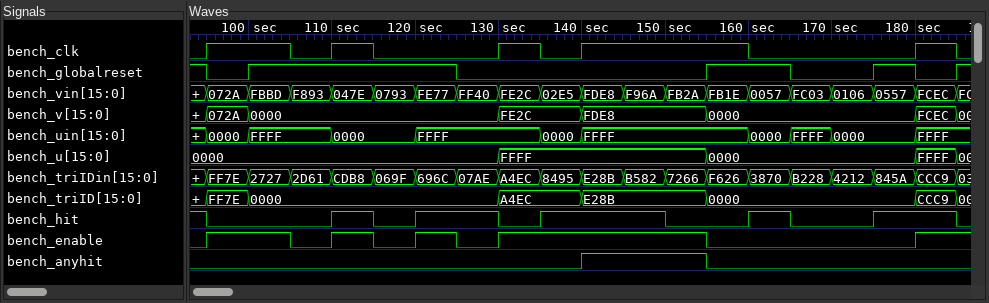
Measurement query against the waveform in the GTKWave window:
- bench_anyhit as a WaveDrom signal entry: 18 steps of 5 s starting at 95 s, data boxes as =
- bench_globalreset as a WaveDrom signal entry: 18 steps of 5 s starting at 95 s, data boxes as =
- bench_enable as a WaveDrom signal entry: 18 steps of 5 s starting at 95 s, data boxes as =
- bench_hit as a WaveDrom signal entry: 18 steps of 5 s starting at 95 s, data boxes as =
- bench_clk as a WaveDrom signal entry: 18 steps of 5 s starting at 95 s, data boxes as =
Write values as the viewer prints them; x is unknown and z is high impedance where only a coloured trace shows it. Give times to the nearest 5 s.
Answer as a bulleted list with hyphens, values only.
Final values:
- {name: 'bench_anyhit', wave: '0........1..0.....'}
- {name: 'bench_globalreset', wave: '01....0.....1.0.10'}
- {name: 'bench_enable', wave: '1.010101....0....1'}
- {name: 'bench_hit', wave: '0..101.01..0.10.1.'}
- {name: 'bench_clk', wave: '1.010..101...0...1'}
